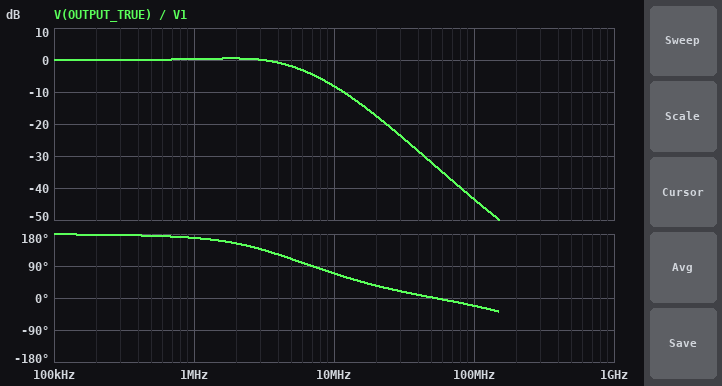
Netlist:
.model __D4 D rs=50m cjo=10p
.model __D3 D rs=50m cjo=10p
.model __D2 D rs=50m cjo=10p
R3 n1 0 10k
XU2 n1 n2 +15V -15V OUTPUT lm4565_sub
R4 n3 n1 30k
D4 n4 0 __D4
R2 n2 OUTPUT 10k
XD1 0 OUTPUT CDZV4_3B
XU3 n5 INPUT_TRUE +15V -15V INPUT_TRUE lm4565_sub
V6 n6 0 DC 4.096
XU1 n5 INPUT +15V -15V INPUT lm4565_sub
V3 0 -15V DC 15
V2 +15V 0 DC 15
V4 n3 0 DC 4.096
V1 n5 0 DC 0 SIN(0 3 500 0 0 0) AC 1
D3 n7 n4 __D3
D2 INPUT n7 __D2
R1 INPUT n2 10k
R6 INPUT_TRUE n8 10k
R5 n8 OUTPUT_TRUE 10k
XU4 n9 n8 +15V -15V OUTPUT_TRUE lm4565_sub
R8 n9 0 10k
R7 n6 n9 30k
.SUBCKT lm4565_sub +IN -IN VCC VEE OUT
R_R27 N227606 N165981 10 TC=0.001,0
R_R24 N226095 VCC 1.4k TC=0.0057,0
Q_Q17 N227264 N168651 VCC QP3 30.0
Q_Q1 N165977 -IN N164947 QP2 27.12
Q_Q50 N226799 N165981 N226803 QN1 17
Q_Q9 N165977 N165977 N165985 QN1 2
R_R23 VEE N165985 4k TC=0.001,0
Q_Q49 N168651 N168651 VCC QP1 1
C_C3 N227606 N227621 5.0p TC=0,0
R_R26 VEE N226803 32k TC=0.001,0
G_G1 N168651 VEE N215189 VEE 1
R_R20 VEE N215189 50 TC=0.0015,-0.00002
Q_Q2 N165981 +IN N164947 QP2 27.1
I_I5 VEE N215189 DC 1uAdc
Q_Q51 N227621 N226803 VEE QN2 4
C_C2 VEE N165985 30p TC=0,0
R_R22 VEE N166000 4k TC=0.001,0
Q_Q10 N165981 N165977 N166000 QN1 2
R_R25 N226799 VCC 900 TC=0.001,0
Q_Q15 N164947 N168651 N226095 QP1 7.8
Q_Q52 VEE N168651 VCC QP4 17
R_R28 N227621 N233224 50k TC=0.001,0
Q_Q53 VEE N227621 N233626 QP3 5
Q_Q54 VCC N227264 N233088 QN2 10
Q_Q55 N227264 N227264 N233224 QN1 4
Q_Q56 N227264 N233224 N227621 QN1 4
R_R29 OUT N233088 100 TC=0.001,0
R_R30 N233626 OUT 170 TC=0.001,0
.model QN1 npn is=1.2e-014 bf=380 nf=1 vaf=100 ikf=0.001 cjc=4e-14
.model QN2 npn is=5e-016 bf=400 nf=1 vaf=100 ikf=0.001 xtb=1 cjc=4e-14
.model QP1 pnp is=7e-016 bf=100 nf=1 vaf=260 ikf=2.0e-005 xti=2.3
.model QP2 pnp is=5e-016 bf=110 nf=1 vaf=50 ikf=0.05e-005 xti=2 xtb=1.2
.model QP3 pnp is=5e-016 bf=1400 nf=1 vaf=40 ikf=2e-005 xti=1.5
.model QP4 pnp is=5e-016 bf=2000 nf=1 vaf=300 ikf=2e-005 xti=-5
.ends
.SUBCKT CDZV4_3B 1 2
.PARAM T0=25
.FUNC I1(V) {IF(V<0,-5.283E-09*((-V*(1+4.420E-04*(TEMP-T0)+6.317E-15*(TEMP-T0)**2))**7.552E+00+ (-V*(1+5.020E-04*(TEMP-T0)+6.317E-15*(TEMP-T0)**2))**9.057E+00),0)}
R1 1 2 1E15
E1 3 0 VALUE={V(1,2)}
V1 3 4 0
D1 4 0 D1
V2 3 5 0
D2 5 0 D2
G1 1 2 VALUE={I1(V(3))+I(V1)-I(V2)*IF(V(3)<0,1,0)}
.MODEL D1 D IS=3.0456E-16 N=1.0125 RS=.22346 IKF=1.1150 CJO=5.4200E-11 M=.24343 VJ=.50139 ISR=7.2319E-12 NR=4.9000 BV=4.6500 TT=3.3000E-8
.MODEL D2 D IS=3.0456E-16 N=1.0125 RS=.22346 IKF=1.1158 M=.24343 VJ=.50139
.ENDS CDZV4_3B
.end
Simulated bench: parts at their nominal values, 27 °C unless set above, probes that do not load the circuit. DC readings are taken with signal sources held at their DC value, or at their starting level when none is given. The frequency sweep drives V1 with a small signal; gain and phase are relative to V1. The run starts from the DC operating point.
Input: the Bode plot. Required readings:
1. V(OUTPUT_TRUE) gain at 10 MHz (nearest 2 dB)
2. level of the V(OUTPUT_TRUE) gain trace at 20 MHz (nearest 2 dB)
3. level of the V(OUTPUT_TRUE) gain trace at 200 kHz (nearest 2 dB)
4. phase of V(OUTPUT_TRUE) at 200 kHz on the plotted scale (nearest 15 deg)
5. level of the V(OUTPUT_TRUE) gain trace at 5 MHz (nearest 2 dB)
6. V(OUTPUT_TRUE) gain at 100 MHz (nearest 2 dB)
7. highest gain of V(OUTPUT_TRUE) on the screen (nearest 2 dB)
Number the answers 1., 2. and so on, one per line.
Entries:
1. -8 dB
2. -18 dB
3. 0 dB
4. 180 deg
5. -2 dB
6. -44 dB
7. 0 dB
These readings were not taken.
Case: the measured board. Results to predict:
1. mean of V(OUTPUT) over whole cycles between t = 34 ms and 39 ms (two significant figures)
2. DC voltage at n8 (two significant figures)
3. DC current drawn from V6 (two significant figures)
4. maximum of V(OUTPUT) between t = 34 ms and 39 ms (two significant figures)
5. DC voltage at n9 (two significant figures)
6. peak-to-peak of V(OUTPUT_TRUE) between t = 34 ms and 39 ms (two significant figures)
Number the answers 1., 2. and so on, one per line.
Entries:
1. 2.1 V
2. 1.0 V
3. 100 µA
4. 4.8 V
5. 1.0 V
6. 6.0 V
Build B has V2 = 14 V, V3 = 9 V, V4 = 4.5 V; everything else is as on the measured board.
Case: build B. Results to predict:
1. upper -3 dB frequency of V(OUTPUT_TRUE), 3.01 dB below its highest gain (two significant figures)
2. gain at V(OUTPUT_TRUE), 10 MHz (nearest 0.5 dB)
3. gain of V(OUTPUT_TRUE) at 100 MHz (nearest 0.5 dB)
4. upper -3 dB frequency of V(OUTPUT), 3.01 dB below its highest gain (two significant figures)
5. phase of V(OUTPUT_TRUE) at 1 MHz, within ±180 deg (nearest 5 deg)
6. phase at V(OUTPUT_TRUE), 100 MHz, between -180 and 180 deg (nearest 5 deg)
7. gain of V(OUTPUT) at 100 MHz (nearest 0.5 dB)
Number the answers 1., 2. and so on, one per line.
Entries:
1. 5.3 MHz
2. -8.5 dB
3. -44.0 dB
4. 6.5 MHz
5. 170 deg
6. -25 deg
7. -63.5 dB
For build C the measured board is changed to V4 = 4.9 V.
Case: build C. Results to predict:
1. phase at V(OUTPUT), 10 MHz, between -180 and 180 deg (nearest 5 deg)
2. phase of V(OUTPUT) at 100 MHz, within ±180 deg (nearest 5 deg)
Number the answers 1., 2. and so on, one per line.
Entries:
1. 35 deg
2. -150 deg
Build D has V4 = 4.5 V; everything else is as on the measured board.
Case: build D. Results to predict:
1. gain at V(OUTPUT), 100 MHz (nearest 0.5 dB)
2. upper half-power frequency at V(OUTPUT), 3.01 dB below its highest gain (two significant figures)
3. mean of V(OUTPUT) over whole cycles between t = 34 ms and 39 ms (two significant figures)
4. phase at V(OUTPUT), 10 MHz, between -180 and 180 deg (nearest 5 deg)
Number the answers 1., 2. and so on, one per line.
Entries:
1. -63.0 dB
2. 6.7 MHz
3. 2.3 V
4. 30 deg
